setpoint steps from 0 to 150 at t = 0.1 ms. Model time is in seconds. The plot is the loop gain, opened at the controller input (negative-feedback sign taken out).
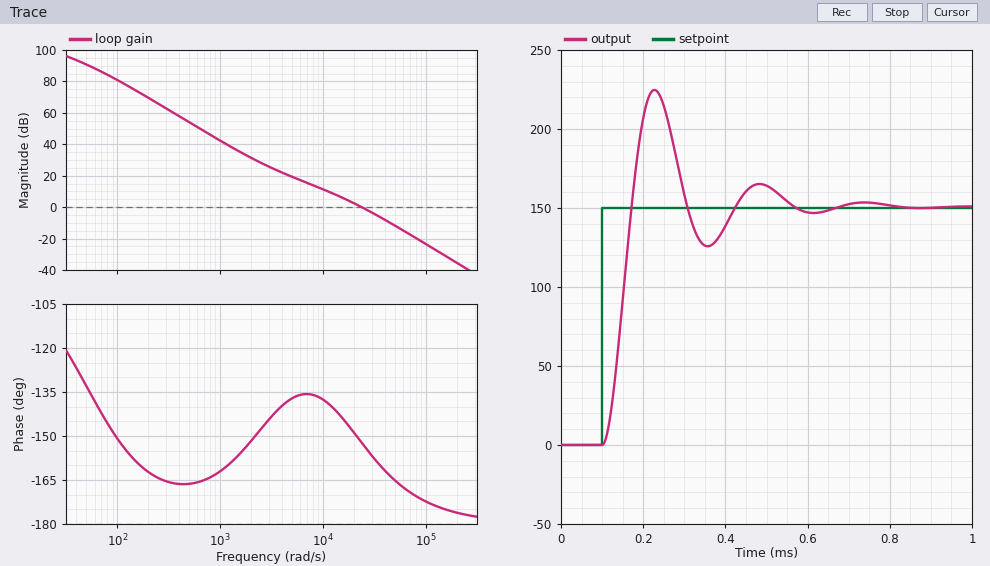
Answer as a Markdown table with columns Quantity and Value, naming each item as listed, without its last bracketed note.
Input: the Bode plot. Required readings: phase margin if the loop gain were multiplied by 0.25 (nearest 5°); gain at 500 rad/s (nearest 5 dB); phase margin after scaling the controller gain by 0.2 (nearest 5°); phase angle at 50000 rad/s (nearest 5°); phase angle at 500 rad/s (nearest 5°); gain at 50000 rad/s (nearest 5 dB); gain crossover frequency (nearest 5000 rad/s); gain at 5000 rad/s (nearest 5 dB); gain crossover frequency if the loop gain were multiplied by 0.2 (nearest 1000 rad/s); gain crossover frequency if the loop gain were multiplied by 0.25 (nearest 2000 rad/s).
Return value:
| Quantity | Value |
|---|---|
| phase margin if the loop gain were multiplied by 0.25 | 45° |
| gain at 500 rad/s | 55 dB |
| phase margin after scaling the controller gain by 0.2 | 45° |
| phase angle at 50000 rad/s | -165° |
| phase angle at 500 rad/s | -165° |
| gain at 50000 rad/s | -10 dB |
| gain crossover frequency | 25000 rad/s |
| gain at 5000 rad/s | 20 dB |
| gain crossover frequency if the loop gain were multiplied by 0.2 | 8000 rad/s |
| gain crossover frequency if the loop gain were multiplied by 0.25 | 10000 rad/s |
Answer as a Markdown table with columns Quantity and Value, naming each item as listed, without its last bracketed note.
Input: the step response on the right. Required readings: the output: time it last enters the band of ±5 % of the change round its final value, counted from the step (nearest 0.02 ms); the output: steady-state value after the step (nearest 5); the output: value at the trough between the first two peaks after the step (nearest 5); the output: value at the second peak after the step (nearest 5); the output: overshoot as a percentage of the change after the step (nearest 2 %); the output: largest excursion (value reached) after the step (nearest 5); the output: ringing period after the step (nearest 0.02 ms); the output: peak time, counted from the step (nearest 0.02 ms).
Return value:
| Quantity | Value |
|---|---|
| the output: time it last enters the band of ±5 % of the change round its final value, counted from the step | 0.44 ms |
| the output: steady-state value after the step | 150 |
| the output: value at the trough between the first two peaks after the step | 125 |
| the output: value at the second peak after the step | 165 |
| the output: overshoot as a percentage of the change after the step | 50 % |
| the output: largest excursion (value reached) after the step | 225 |
| the output: ringing period after the step | 0.26 ms |
| the output: peak time, counted from the step | 0.12 ms |
